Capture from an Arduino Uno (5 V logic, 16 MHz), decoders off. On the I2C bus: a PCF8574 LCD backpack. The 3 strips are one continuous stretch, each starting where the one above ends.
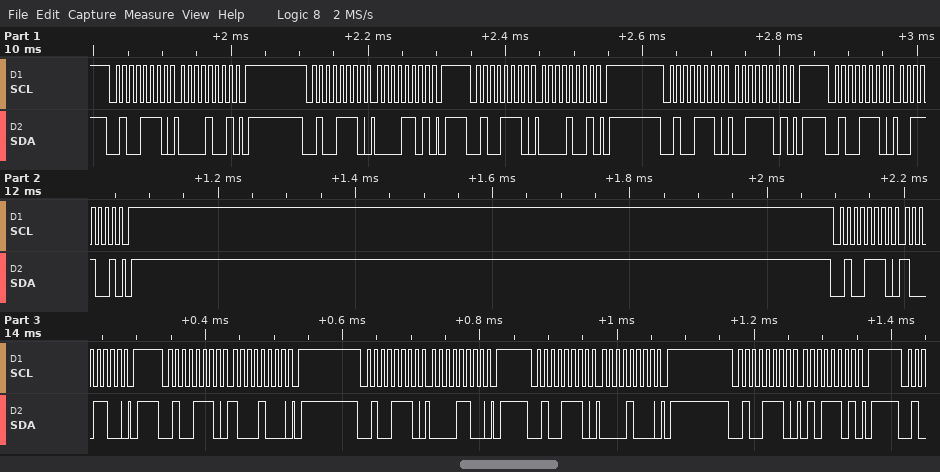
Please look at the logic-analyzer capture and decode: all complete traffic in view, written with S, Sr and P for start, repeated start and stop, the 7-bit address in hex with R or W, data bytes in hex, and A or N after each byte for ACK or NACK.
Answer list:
S 27W A 09 A P S 27W A 0D A P S 27W A 09 A P S 27W A 3D A P S 27W A 39 A P S 27W A 8C A P S 27W A 88 A P S 27W A 0C A P S 27W A 08 A P S 27W A 5D A P
